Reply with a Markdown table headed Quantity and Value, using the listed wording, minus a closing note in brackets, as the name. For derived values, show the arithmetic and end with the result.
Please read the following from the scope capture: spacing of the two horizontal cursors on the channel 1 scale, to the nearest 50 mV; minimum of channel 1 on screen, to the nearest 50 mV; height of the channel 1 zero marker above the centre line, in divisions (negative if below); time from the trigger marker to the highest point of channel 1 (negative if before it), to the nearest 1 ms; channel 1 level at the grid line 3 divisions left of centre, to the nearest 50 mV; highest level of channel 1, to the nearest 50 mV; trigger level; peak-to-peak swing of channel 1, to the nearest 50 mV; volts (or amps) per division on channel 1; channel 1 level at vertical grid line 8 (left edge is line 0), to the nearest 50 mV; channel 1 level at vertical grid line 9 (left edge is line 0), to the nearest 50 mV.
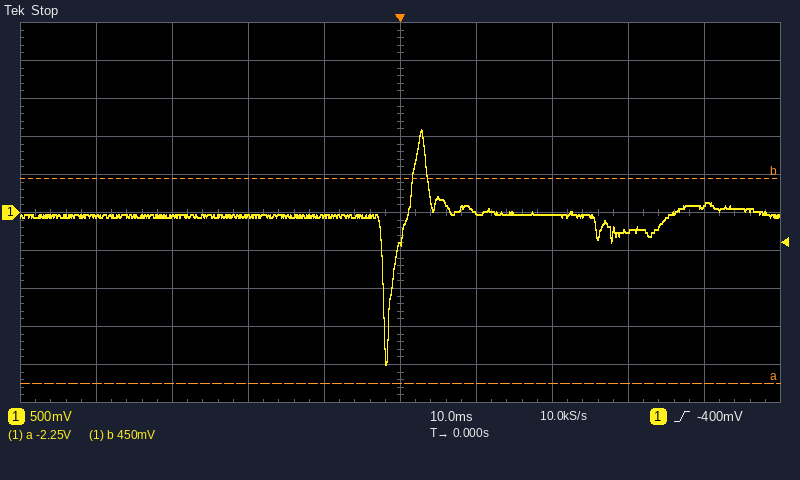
| Quantity | Value |
|---|---|
| spacing of the two horizontal cursors on the channel 1 scale, to the nearest 50 mV | 2.70 V |
| minimum of channel 1 on screen, to the nearest 50 mV | -2.00 V |
| height of the channel 1 zero marker above the centre line, in divisions | 0.0 div |
| time from the trigger marker to the highest point of channel 1 (negative if before it), to the nearest 1 ms | +3 ms |
| channel 1 level at the grid line 3 divisions left of centre, to the nearest 50 mV | -50 mV |
| highest level of channel 1, to the nearest 50 mV | 1.10 V |
| trigger level | -400 mV |
| peak-to-peak swing of channel 1, to the nearest 50 mV | 1.10 V − (-2.00 V) = 3.10 V |
| volts (or amps) per division on channel 1 | 500 mV |
| channel 1 level at vertical grid line 8 (left edge is line 0), to the nearest 50 mV | -250 mV |
| channel 1 level at vertical grid line 9 (left edge is line 0), to the nearest 50 mV | 100 mV |
